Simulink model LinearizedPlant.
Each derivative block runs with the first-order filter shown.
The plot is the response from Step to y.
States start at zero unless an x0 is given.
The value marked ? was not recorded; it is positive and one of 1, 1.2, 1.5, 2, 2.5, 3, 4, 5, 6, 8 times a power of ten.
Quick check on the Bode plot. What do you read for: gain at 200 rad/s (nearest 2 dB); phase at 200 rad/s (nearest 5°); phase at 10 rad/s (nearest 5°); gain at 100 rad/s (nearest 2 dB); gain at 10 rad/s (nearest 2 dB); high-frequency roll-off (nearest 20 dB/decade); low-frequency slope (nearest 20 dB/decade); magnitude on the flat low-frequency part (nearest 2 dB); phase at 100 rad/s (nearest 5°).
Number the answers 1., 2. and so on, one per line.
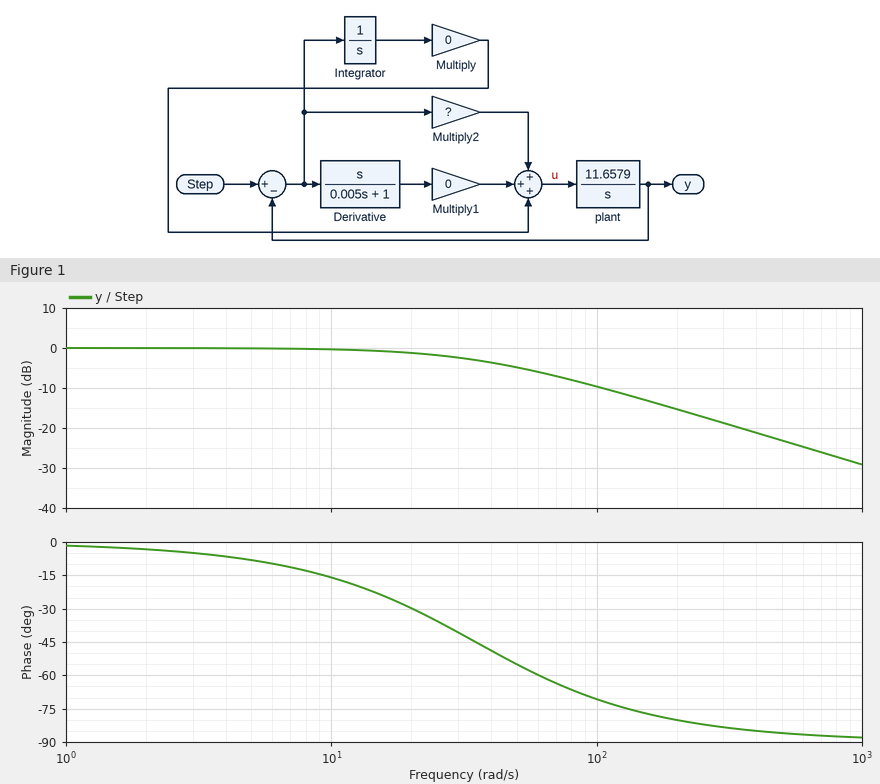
1. -16 dB
2. -80°
3. -15°
4. -10 dB
5. 0 dB
6. -20 dB/decade
7. 0 dB/decade
8. 0 dB
9. -70°
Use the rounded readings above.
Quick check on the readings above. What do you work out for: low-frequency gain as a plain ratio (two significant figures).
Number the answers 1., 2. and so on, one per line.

1. 1.0
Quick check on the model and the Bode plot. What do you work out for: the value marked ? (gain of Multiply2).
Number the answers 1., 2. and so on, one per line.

1. 3
